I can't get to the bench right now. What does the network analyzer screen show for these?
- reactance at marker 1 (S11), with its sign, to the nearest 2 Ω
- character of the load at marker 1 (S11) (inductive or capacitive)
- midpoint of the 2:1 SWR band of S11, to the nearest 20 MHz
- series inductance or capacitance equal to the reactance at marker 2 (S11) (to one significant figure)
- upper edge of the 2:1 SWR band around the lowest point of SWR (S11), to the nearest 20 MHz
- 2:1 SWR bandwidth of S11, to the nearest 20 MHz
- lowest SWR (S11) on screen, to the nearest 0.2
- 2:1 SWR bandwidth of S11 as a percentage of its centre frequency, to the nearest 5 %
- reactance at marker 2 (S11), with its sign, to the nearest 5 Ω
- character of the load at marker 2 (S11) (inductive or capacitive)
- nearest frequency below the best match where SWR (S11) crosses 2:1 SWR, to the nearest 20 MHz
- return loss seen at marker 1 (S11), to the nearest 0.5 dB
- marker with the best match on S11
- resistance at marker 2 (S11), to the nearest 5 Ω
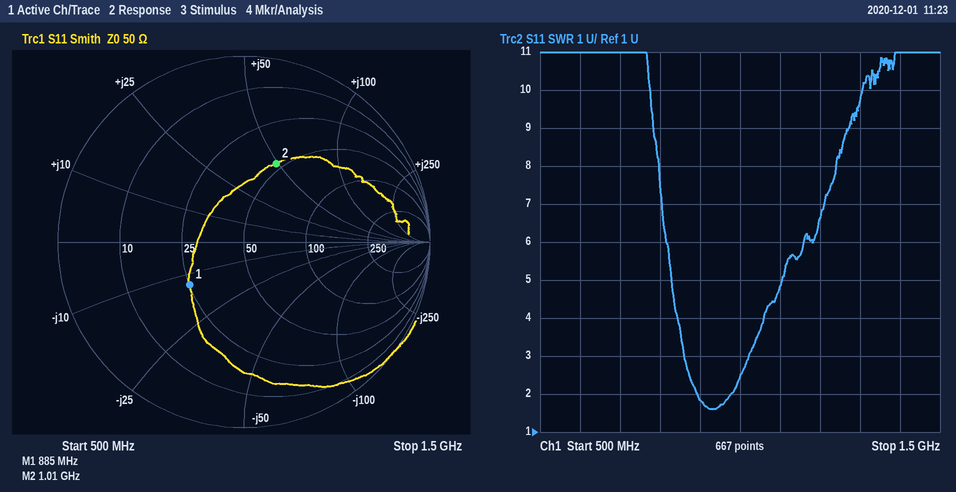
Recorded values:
-14 Ω
capacitive
940 MHz
8 nH
980 MHz
80 MHz
1.6
10 %
+50 Ω
inductive
900 MHz
8.5 dB
marker 1
45 Ω
